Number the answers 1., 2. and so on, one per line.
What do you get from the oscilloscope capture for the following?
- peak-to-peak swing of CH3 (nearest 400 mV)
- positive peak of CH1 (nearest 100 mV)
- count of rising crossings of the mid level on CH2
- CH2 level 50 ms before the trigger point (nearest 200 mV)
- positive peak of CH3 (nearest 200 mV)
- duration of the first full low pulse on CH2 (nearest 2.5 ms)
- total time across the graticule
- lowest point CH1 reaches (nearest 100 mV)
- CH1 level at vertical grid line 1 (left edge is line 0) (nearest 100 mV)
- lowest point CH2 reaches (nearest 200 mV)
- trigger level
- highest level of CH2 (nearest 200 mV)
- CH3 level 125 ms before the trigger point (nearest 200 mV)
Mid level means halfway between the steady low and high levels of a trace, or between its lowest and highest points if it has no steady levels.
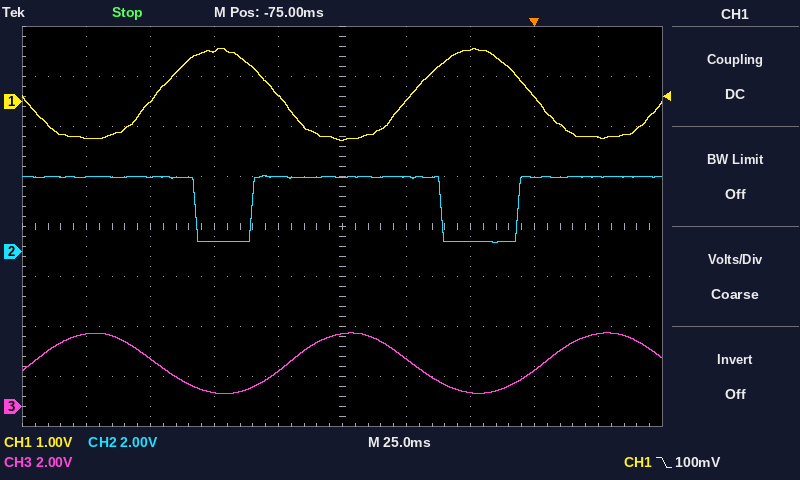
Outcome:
1. 2.4 V
2. 1.1 V
3. 2
4. 3.0 V
5. 3.0 V
6. 22.5 ms
7. 250 ms
8. -800 mV
9. -700 mV
10. 400 mV
11. 100 mV
12. 3.0 V
13. 600 mV
